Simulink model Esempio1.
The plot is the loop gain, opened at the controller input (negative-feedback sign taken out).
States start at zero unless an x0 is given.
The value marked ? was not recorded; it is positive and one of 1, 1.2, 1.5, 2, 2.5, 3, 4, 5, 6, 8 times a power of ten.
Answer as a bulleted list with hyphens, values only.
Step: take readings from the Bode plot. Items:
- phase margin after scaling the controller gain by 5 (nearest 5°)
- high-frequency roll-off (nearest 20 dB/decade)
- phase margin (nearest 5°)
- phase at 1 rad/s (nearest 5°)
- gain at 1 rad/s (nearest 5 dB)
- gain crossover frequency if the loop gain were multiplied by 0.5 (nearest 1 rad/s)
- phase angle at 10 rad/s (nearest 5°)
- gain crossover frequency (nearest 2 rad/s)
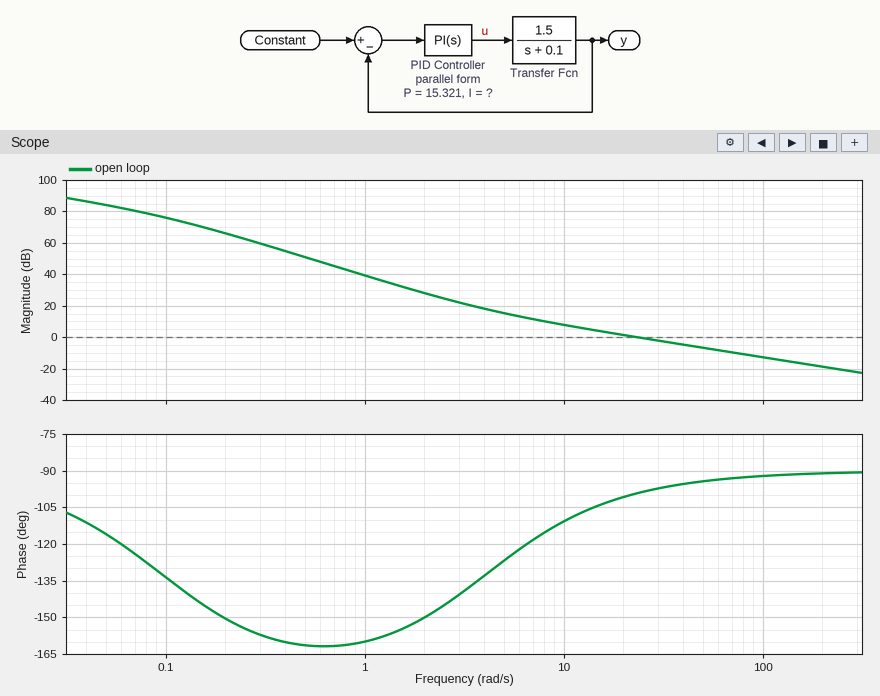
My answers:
- 90°
- -20 dB/decade
- 80°
- -160°
- 40 dB
- 12 rad/s
- -110°
- 24 rad/s
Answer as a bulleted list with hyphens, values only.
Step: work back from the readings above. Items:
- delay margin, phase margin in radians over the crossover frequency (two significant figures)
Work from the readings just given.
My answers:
- 0.058 s
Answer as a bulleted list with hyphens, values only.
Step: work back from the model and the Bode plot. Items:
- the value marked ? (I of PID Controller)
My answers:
- 60
